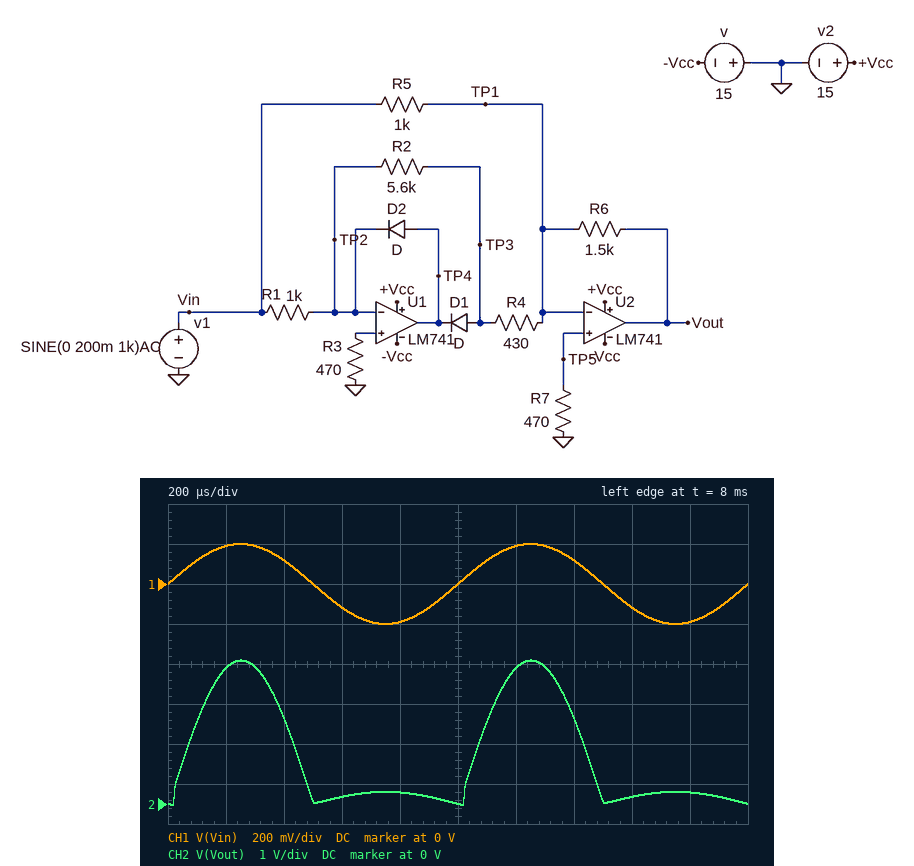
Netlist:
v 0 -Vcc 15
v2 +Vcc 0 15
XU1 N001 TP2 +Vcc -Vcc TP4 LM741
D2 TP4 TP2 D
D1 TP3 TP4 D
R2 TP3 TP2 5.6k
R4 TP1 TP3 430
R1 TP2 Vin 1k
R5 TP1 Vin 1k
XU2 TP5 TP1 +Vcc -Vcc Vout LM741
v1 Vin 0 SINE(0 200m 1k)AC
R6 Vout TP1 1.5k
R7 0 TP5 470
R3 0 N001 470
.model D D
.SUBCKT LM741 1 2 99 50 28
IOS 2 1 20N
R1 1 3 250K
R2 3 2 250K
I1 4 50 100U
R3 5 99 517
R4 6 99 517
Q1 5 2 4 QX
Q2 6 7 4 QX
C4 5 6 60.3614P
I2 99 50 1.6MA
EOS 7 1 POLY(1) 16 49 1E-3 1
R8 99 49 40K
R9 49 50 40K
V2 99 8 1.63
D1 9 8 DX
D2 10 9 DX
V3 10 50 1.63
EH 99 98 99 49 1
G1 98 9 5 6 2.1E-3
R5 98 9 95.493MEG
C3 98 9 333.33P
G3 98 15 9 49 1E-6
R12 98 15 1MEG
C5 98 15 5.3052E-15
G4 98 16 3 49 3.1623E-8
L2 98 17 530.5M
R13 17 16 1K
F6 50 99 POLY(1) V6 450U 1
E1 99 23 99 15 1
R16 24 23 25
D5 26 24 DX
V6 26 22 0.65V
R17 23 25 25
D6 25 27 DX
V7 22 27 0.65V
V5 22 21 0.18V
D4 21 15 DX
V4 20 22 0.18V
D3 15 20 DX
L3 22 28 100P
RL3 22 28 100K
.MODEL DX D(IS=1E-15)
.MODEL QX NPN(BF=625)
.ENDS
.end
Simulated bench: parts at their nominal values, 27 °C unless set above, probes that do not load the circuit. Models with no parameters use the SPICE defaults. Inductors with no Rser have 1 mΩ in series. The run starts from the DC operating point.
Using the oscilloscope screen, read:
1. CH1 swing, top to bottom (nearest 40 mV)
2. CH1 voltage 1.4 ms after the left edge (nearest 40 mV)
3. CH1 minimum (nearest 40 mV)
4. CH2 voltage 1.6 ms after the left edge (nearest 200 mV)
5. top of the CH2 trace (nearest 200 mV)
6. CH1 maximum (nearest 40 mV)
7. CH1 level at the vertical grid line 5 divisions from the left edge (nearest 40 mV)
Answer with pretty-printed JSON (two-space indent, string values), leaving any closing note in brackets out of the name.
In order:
{
  "CH1 swing, top to bottom": "400 mV",
  "CH1 voltage 1.4 ms after the left edge": "120 mV",
  "CH1 minimum": "-200 mV",
  "CH2 voltage 1.6 ms after the left edge": "200 mV",
  "top of the CH2 trace": "3.6 V",
  "CH1 maximum": "200 mV",
  "CH1 level at the vertical grid line 5 divisions from the left edge": "0 V"
}
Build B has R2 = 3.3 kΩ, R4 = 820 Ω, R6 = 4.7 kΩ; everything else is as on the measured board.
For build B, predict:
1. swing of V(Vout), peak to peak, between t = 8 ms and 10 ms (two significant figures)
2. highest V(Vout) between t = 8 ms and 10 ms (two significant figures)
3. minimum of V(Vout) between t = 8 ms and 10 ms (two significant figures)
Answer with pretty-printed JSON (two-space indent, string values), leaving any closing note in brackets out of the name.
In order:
{
  "swing of V(Vout), peak to peak, between t = 8 ms and 10 ms": "2.9 V",
  "highest V(Vout) between t = 8 ms and 10 ms": "2.8 V",
  "minimum of V(Vout) between t = 8 ms and 10 ms": "-110 mV"
}
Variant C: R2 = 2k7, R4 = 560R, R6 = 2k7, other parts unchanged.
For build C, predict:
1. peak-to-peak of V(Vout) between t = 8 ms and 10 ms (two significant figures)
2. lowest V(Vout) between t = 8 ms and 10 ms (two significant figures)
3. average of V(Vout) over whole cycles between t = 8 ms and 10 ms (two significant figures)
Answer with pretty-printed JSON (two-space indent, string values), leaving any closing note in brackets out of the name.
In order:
{
  "peak-to-peak of V(Vout) between t = 8 ms and 10 ms": "2.1 V",
  "lowest V(Vout) between t = 8 ms and 10 ms": "-70 mV",
  "average of V(Vout) over whole cycles between t = 8 ms and 10 ms": "820 mV"
}
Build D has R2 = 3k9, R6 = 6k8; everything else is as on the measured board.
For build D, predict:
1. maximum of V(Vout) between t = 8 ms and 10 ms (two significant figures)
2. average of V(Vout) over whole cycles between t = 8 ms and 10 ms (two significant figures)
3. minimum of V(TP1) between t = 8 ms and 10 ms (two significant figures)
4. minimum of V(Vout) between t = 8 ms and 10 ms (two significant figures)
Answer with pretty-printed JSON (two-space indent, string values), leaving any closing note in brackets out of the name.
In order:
{
  "maximum of V(Vout) between t = 8 ms and 10 ms": "11 V",
  "average of V(Vout) over whole cycles between t = 8 ms and 10 ms": "3.9 V",
  "minimum of V(TP1) between t = 8 ms and 10 ms": "-37 mV",
  "minimum of V(Vout) between t = 8 ms and 10 ms": "-160 mV"
}
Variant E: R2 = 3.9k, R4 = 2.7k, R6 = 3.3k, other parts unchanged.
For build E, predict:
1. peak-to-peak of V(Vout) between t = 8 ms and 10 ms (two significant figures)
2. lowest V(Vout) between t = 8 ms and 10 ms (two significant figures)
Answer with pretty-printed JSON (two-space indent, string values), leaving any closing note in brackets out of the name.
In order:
{
  "peak-to-peak of V(Vout) between t = 8 ms and 10 ms": "740 mV",
  "lowest V(Vout) between t = 8 ms and 10 ms": "-74 mV"
}
